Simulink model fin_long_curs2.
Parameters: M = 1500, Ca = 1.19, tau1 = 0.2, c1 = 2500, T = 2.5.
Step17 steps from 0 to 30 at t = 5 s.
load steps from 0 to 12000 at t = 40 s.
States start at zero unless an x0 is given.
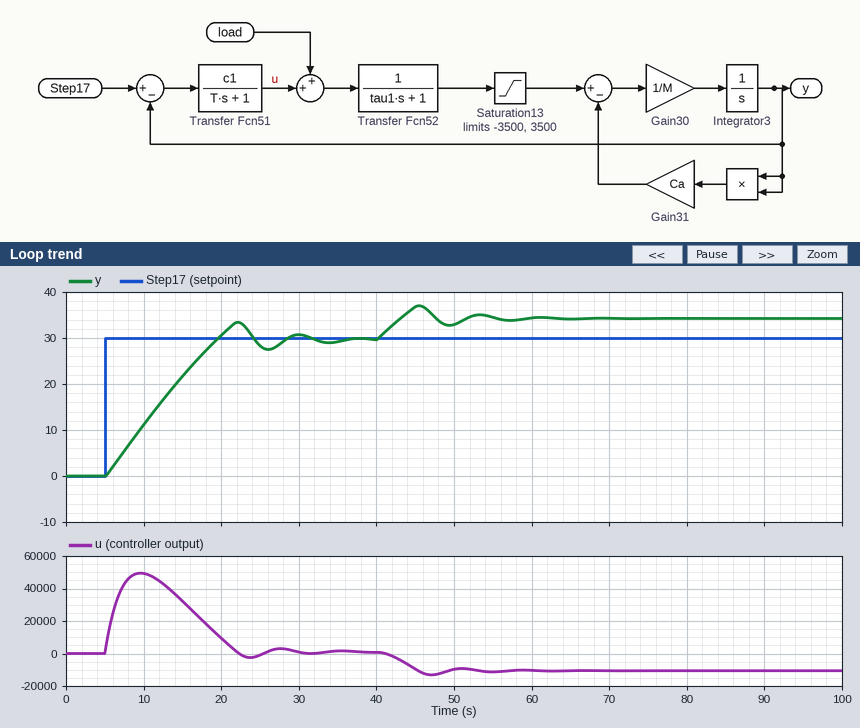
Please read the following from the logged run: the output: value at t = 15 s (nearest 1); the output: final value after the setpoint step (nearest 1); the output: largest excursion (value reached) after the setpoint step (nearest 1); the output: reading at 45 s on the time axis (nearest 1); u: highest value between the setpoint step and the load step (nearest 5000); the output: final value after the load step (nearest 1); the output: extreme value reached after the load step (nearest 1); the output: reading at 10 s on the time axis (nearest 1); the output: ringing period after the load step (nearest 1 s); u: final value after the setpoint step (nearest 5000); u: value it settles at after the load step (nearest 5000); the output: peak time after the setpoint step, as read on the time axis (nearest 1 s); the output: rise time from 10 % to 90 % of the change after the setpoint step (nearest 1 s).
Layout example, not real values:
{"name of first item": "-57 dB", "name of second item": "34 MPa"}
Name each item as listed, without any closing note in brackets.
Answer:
{"the output: value at t = 15 s": "22", "the output: final value after the setpoint step": "30", "the output: largest excursion (value reached) after the setpoint step": "33", "the output: reading at 45 s on the time axis": "37", "u: highest value between the setpoint step and the load step": "50000", "the output: final value after the load step": "34", "the output: extreme value reached after the load step": "37", "the output: reading at 10 s on the time axis": "11", "the output: ringing period after the load step": "8 s", "u: final value after the setpoint step": "0", "u: value it settles at after the load step": "-10000", "the output: peak time after the setpoint step, as read on the time axis": "22 s", "the output: rise time from 10 % to 90 % of the change after the setpoint step": "11 s"}
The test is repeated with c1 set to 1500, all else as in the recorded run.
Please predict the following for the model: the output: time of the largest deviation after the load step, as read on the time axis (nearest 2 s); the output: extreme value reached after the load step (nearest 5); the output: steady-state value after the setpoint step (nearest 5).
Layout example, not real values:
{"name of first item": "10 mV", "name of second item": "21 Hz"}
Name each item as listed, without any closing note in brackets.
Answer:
{"the output: time of the largest deviation after the load step, as read on the time axis": "48 s", "the output: extreme value reached after the load step": "40", "the output: steady-state value after the setpoint step": "30"}
